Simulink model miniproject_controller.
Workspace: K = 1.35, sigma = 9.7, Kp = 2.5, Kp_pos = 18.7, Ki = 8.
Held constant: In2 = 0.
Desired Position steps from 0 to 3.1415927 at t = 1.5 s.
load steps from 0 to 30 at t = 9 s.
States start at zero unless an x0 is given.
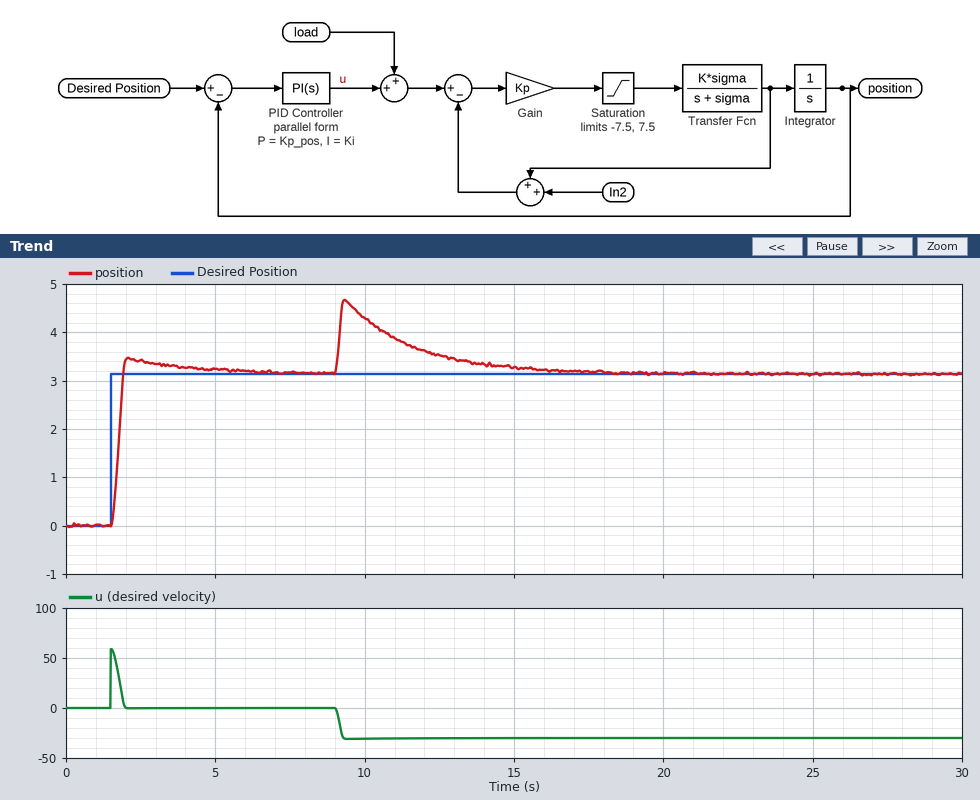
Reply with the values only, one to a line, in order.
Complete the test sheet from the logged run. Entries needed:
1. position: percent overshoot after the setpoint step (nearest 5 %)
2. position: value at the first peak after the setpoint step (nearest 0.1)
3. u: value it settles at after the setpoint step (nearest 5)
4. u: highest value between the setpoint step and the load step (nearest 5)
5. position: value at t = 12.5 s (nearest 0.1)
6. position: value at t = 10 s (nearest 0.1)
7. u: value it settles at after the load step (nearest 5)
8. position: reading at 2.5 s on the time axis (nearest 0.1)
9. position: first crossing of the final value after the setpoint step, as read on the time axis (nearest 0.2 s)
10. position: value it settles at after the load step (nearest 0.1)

10 %
3.5
0
60
3.5
4.3
-30
3.4
2.0 s
3.1
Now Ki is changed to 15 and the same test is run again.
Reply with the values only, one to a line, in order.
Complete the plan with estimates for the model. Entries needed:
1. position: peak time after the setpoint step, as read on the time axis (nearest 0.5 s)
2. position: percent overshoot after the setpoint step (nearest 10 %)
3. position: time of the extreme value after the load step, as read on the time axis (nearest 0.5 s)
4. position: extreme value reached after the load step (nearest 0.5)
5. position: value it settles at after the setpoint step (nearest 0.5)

2.0 s
20 %
9.5 s
4.5
3.0
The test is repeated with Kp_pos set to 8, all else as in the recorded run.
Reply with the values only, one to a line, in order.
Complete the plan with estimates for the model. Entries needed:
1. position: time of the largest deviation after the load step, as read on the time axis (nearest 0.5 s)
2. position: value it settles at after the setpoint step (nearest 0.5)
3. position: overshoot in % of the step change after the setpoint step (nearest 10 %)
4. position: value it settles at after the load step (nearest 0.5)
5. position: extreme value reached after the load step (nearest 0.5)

9.5 s
3.0
20 %
3.0
6.0
